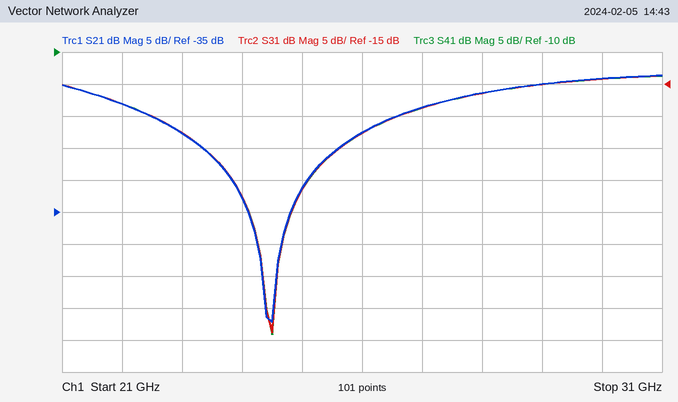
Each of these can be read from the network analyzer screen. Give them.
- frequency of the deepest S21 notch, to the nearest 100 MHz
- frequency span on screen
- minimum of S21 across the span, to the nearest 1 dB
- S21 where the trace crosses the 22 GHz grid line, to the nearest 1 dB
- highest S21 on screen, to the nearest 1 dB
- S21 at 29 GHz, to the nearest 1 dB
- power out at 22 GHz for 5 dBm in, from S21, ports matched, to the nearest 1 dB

24.5 GHz
10 GHz
-52 dB
-18 dB
-14 dB
-15 dB
-13 dBm
